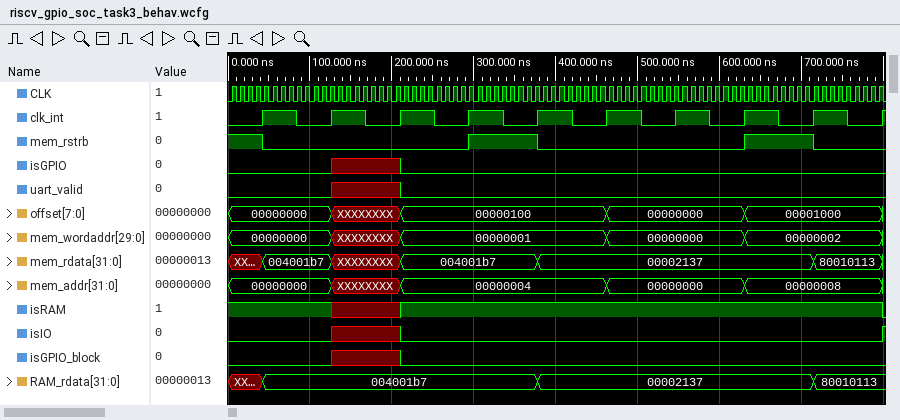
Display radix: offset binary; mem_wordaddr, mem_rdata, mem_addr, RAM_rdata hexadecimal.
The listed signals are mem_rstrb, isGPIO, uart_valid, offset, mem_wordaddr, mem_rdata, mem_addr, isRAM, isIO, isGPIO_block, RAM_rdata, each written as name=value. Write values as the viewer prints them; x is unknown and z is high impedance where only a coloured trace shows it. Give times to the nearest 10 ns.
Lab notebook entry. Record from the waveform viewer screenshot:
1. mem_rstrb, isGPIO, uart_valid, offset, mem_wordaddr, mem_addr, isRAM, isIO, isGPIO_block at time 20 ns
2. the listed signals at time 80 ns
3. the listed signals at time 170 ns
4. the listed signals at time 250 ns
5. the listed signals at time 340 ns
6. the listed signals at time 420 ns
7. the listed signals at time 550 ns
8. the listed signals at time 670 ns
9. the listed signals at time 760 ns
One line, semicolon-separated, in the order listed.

mem_rstrb=1, isGPIO=0, uart_valid=0, offset=00000000, mem_wordaddr=00000000, mem_addr=00000000, isRAM=1, isIO=0, isGPIO_block=0; mem_rstrb=0, isGPIO=0, uart_valid=0, offset=00000000, mem_wordaddr=00000000, mem_rdata=004001b7, mem_addr=00000000, isRAM=1, isIO=0, isGPIO_block=0, RAM_rdata=004001b7; mem_rstrb=0, isGPIO=x, uart_valid=x, offset=XXXXXXXX, mem_wordaddr=XXXXXXXX, mem_rdata=XXXXXXXX, mem_addr=XXXXXXXX, isRAM=x, isIO=x, isGPIO_block=x, RAM_rdata=004001b7; mem_rstrb=0, isGPIO=0, uart_valid=0, offset=00000100, mem_wordaddr=00000001, mem_rdata=004001b7, mem_addr=00000004, isRAM=1, isIO=0, isGPIO_block=0, RAM_rdata=004001b7; mem_rstrb=1, isGPIO=0, uart_valid=0, offset=00000100, mem_wordaddr=00000001, mem_rdata=004001b7, mem_addr=00000004, isRAM=1, isIO=0, isGPIO_block=0, RAM_rdata=004001b7; mem_rstrb=0, isGPIO=0, uart_valid=0, offset=00000100, mem_wordaddr=00000001, mem_rdata=00002137, mem_addr=00000004, isRAM=1, isIO=0, isGPIO_block=0, RAM_rdata=00002137; mem_rstrb=0, isGPIO=0, uart_valid=0, offset=00000000, mem_wordaddr=00000000, mem_rdata=00002137, mem_addr=00000000, isRAM=1, isIO=0, isGPIO_block=0, RAM_rdata=00002137; mem_rstrb=1, isGPIO=0, uart_valid=0, offset=00001000, mem_wordaddr=00000002, mem_rdata=00002137, mem_addr=00000008, isRAM=1, isIO=0, isGPIO_block=0, RAM_rdata=00002137; mem_rstrb=0, isGPIO=0, uart_valid=0, offset=00001000, mem_wordaddr=00000002, mem_rdata=80010113, mem_addr=00000008, isRAM=1, isIO=0, isGPIO_block=0, RAM_rdata=80010113
